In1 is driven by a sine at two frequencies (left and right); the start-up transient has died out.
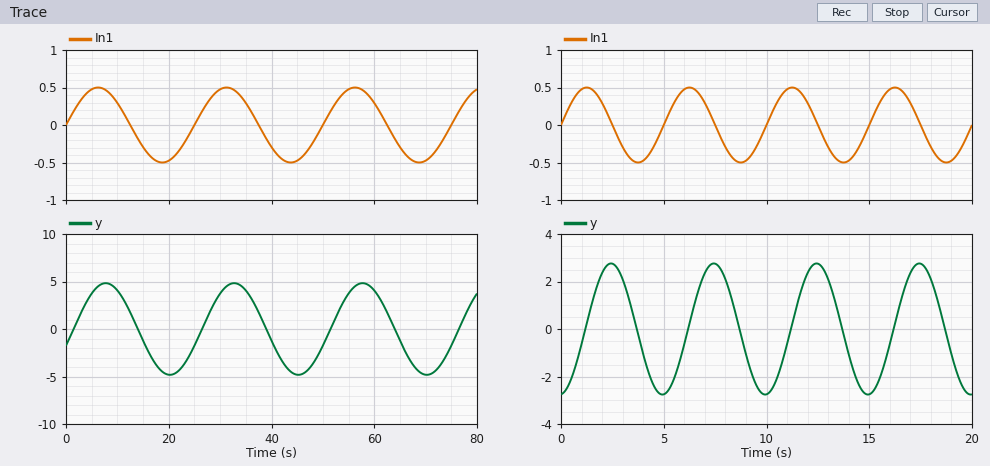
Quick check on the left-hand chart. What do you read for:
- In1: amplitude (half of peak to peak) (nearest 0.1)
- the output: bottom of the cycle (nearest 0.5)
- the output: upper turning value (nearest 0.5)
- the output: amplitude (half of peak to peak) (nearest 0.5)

0.5
-5.0
5.0
5.0
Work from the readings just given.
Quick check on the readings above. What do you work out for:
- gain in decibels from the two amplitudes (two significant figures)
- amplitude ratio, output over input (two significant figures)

20 dB
10
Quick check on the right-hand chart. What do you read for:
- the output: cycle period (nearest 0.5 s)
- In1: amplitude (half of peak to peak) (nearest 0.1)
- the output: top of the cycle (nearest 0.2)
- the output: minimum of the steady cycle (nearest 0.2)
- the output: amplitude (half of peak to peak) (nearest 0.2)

5.0 s
0.5
2.8
-2.8
2.8
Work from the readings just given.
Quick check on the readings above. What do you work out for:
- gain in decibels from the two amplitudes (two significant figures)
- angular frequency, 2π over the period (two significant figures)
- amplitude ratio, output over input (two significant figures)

15 dB
1.3 rad/s
5.6
